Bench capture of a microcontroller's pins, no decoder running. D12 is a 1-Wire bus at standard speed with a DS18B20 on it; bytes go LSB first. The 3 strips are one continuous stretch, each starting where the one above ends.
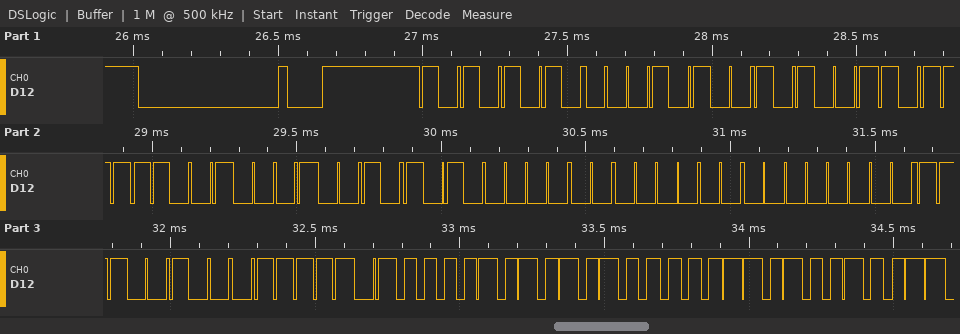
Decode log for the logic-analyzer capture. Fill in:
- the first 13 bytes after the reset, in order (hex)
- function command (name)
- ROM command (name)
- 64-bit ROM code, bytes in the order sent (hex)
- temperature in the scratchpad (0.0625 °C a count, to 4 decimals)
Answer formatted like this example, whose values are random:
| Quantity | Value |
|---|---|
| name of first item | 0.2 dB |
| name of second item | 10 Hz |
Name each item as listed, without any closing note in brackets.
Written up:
| Quantity | Value |
|---|---|
| the first 13 bytes after the reset, in order | 55 28 65 9F 48 05 00 00 27 BE 50 05 4B |
| function command | Read Scratchpad |
| ROM command | Match ROM |
| 64-bit ROM code, bytes in the order sent | 28 65 9F 48 05 00 00 27 |
| temperature in the scratchpad | 85.0000 °C |
